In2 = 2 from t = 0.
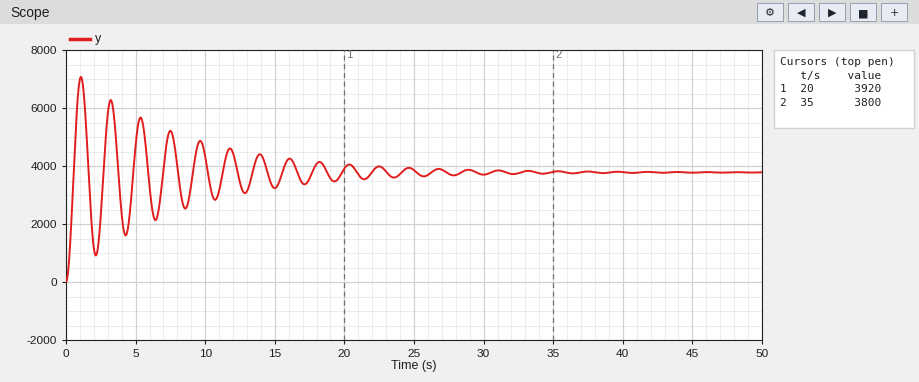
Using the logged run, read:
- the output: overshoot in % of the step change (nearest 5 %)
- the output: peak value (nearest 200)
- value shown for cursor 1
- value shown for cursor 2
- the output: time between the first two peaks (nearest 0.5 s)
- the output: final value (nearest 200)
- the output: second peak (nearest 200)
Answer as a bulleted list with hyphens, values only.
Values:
- 85 %
- 7000
- 3920
- 3800
- 2.0 s
- 3800
- 6200
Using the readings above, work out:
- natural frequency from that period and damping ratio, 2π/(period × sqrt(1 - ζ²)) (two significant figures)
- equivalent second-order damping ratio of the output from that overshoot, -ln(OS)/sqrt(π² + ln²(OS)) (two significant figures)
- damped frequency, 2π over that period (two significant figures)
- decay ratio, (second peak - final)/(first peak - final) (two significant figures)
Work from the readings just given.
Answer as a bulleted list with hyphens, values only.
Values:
- 3.1 rad/s
- 0.052
- 3.1 rad/s
- 0.75
